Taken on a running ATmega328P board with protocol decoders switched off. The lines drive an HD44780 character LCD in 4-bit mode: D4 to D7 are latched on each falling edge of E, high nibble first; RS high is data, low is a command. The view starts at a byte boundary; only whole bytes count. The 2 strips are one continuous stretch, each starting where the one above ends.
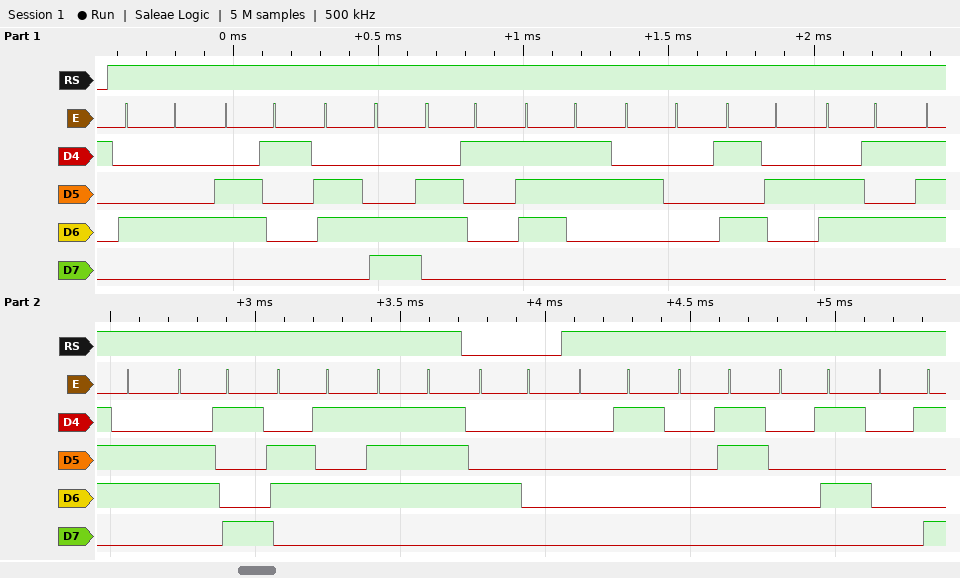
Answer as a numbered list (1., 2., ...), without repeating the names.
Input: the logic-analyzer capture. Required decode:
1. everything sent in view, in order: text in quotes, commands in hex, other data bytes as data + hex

1. "Dalas Review" 0x40 data 01 03 05 09
